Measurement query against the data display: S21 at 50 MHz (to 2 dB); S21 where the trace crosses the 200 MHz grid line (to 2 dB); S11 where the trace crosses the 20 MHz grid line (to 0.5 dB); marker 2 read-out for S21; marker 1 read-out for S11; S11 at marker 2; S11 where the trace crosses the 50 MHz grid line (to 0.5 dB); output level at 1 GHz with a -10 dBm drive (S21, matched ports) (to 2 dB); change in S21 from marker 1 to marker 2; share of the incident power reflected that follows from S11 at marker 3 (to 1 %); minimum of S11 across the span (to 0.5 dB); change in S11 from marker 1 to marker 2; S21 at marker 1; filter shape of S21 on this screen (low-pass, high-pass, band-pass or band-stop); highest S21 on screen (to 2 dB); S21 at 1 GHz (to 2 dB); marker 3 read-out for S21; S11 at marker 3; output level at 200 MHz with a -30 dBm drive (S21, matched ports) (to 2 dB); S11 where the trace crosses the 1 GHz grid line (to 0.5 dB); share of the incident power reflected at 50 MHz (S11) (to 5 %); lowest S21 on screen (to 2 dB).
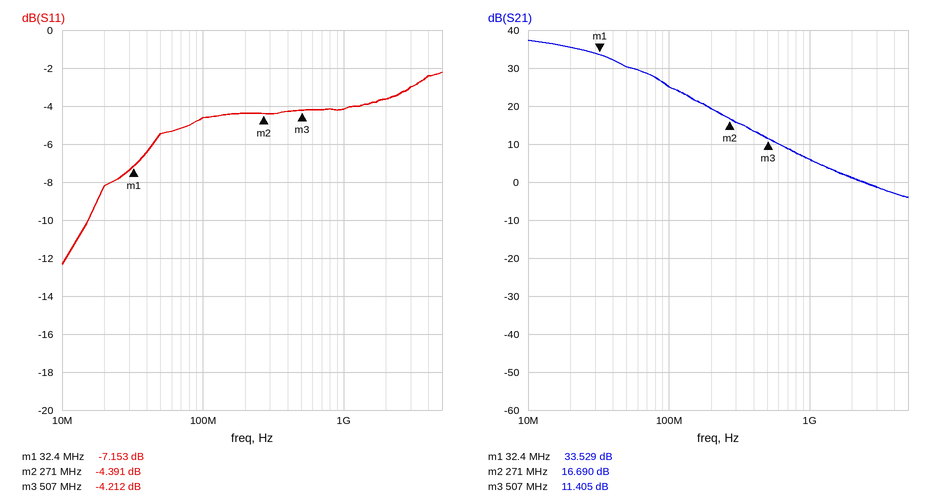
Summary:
30 dB
20 dB
-8.0 dB
16.690 dB
-7.153 dB
-4.391 dB
-5.5 dB
-4 dBm
-16.839 dB
38 %
-12.5 dB
2.762 dB
33.529 dB
low-pass
38 dB
6 dB
11.405 dB
-4.212 dB
-10 dBm
-4.0 dB
30 %
-4 dB
